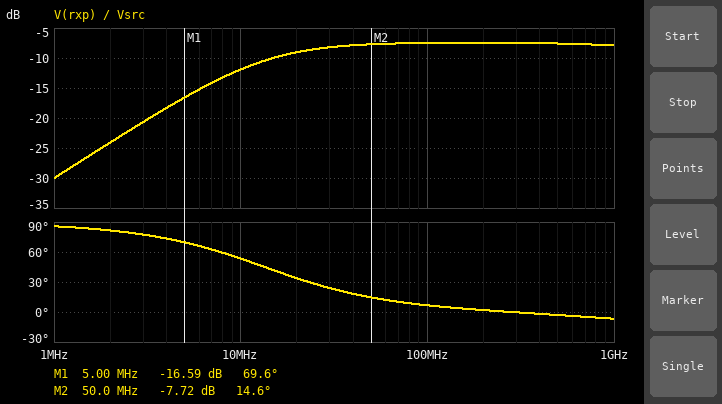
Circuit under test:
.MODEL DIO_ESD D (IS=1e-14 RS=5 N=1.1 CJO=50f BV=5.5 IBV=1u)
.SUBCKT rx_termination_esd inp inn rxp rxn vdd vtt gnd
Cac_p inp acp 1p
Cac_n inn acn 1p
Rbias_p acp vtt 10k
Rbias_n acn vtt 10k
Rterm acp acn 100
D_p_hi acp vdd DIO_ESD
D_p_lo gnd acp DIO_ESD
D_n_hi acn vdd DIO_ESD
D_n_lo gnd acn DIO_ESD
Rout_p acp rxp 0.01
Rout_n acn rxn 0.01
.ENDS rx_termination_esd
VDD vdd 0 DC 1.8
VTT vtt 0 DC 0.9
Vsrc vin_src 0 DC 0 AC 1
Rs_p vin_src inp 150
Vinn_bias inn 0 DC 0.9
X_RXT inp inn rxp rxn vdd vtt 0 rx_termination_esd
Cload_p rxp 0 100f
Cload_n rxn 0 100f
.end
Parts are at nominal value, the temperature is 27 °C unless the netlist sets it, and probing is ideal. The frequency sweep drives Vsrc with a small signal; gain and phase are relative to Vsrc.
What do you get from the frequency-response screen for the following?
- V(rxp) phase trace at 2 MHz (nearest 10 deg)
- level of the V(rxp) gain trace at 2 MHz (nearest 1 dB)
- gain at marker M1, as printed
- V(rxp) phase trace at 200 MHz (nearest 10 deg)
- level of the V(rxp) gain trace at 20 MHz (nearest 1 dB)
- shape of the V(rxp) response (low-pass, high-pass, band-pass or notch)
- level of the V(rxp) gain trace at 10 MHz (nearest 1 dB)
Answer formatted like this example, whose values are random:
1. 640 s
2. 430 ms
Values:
1. 80 deg
2. -24 dB
3. -16.59 dB
4. 0 deg
5. -9 dB
6. high-pass
7. -12 dB
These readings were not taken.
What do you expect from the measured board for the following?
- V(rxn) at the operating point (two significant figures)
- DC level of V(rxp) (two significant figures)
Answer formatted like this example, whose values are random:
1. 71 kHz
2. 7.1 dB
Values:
1. 900 mV
2. 900 mV
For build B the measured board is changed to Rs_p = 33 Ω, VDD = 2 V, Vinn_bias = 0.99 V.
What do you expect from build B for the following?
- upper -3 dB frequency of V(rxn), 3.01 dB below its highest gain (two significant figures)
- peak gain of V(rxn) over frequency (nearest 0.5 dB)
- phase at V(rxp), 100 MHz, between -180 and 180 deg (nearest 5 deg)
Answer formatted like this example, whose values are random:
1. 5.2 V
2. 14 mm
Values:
1. 2.2 GHz
2. -7.5 dB
3. 10 deg
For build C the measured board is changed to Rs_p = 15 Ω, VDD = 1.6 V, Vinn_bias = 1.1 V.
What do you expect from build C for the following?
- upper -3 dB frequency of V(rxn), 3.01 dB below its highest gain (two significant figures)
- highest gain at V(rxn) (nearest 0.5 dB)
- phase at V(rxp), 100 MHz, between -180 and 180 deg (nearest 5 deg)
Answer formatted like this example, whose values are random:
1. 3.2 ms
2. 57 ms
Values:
1. 2.5 GHz
2. -7.5 dB
3. 10 deg
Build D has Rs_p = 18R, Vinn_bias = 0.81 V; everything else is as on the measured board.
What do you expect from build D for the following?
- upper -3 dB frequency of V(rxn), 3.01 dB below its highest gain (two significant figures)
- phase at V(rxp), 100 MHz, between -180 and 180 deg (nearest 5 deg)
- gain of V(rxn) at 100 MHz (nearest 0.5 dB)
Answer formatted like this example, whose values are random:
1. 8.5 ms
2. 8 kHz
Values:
1. 2.4 GHz
2. 10 deg
3. -7.5 dB
